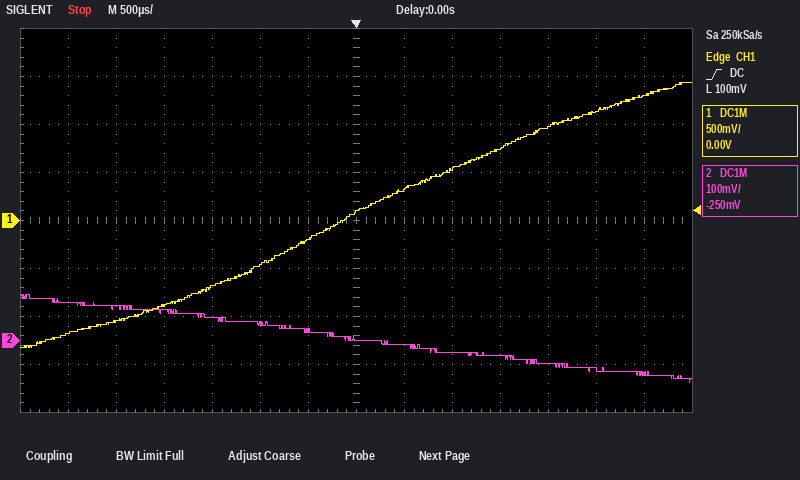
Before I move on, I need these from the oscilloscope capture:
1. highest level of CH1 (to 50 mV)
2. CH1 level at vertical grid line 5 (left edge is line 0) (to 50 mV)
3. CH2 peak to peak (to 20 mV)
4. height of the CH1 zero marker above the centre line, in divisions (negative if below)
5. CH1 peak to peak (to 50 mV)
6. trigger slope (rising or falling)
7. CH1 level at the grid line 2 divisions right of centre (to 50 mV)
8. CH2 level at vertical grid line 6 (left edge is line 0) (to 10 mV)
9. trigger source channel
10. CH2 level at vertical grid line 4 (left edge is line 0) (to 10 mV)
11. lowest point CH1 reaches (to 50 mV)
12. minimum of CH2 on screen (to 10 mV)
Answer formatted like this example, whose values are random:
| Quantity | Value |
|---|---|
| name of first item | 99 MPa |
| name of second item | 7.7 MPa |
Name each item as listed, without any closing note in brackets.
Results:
| Quantity | Value |
|---|---|
| highest level of CH1 | 1.45 V |
| CH1 level at vertical grid line 5 (left edge is line 0) | -450 mV |
| CH2 peak to peak | 180 mV |
| height of the CH1 zero marker above the centre line, in divisions | 0.0 div |
| CH1 peak to peak | 2.75 V |
| trigger slope | rising |
| CH1 level at the grid line 2 divisions right of centre | 550 mV |
| CH2 level at vertical grid line 6 (left edge is line 0) | 20 mV |
| trigger source channel | CH1 |
| CH2 level at vertical grid line 4 (left edge is line 0) | 50 mV |
| lowest point CH1 reaches | -1.30 V |
| minimum of CH2 on screen | -90 mV |
